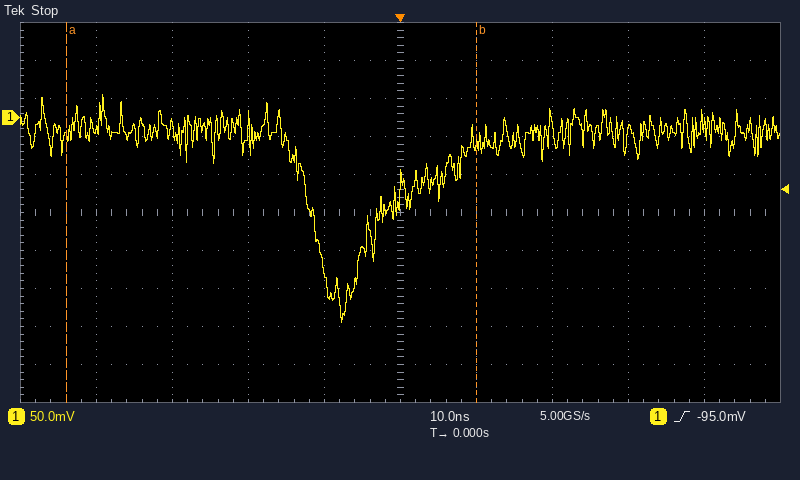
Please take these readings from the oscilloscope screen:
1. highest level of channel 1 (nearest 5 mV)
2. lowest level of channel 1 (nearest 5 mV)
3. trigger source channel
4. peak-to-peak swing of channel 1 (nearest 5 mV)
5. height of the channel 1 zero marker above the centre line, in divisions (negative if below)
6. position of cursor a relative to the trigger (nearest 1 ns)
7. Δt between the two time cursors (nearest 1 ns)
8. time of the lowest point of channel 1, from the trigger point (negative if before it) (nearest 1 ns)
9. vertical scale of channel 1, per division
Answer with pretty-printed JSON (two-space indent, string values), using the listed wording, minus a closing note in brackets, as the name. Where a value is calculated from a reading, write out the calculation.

{
  "highest level of channel 1": "30 mV",
  "lowest level of channel 1": "-270 mV",
  "trigger source channel": "channel 1",
  "peak-to-peak swing of channel 1": "30 mV − (-270 mV) = 300 mV",
  "height of the channel 1 zero marker above the centre line, in divisions": "+2.5 div",
  "position of cursor a relative to the trigger": "-44 ns",
  "Δt between the two time cursors": "54 ns",
  "time of the lowest point of channel 1, from the trigger point (negative if before it)": "-8 ns",
  "vertical scale of channel 1, per division": "50 mV"
}
